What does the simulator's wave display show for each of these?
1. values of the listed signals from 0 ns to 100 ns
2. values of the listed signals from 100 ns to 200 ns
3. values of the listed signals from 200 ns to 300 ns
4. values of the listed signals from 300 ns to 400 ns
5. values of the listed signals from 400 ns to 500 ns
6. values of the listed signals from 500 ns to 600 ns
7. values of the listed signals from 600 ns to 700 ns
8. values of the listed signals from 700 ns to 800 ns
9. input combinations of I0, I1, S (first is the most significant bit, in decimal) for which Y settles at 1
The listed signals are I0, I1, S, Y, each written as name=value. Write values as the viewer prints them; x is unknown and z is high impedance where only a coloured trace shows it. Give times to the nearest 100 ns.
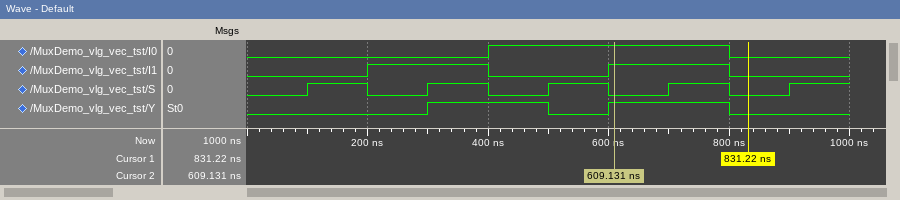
I0=0, I1=0, S=0, Y=0
I0=0, I1=0, S=1, Y=0
I0=0, I1=1, S=0, Y=0
I0=0, I1=1, S=1, Y=1
I0=1, I1=0, S=0, Y=1
I0=1, I1=0, S=1, Y=0
I0=1, I1=1, S=0, Y=1
I0=1, I1=1, S=1, Y=1
3, 4, 6, 7
